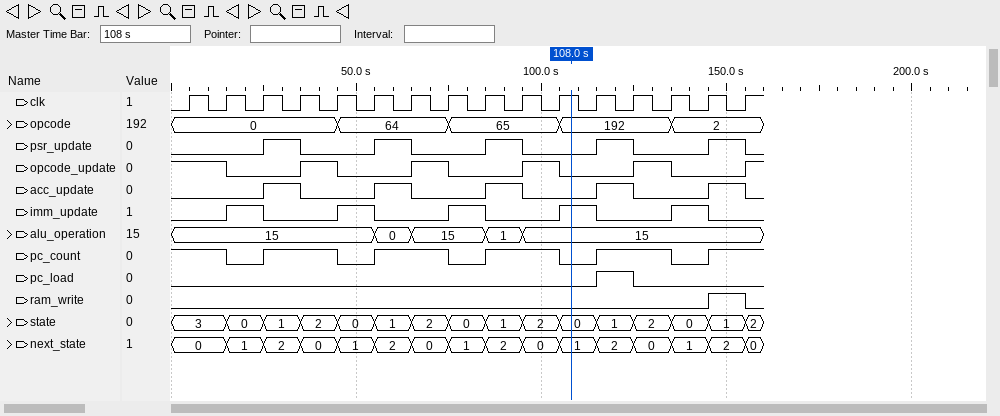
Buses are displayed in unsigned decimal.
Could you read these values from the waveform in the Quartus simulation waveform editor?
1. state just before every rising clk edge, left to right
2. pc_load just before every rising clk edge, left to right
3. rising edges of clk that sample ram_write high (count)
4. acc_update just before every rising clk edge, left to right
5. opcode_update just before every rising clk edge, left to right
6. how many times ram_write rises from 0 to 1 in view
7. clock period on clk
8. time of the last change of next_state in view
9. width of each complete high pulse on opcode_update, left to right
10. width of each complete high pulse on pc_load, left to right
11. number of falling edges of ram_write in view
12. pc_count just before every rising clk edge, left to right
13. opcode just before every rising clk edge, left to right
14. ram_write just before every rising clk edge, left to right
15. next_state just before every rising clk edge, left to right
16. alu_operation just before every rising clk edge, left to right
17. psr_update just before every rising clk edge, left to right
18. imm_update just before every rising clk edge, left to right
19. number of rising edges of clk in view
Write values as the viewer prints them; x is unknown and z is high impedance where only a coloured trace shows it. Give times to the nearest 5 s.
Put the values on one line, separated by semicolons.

3, 3, 0, 1, 2, 0, 1, 2, 0, 1, 2, 0, 1, 2, 0, 1; 0 0 0 0 0 0 0 0 0 0 0 0 1 0 0 0; 1; 0 0 0 1 0 0 1 0 0 1 0 0 1 0 0 1; 1 1 0 0 1 0 0 1 0 0 1 0 0 1 0 0; 1; 10 s; 155 s; 10 s, 10 s, 10 s, 10 s; 10 s; 1; 1 1 0 1 1 0 1 1 0 1 1 0 1 1 0 1; 0, 0, 0, 0, 0, 64, 64, 64, 65, 65, 65, 192, 192, 192, 2, 2; 0 0 0 0 0 0 0 0 0 0 0 0 0 0 0 1; 0, 0, 1, 2, 0, 1, 2, 0, 1, 2, 0, 1, 2, 0, 1, 2; 15, 15, 15, 15, 15, 15, 0, 15, 15, 1, 15, 15, 15, 15, 15, 15; 0 0 0 1 0 0 1 0 0 1 0 0 1 0 0 1; 0 0 1 0 0 1 0 0 1 0 0 1 0 0 1 0; 16
